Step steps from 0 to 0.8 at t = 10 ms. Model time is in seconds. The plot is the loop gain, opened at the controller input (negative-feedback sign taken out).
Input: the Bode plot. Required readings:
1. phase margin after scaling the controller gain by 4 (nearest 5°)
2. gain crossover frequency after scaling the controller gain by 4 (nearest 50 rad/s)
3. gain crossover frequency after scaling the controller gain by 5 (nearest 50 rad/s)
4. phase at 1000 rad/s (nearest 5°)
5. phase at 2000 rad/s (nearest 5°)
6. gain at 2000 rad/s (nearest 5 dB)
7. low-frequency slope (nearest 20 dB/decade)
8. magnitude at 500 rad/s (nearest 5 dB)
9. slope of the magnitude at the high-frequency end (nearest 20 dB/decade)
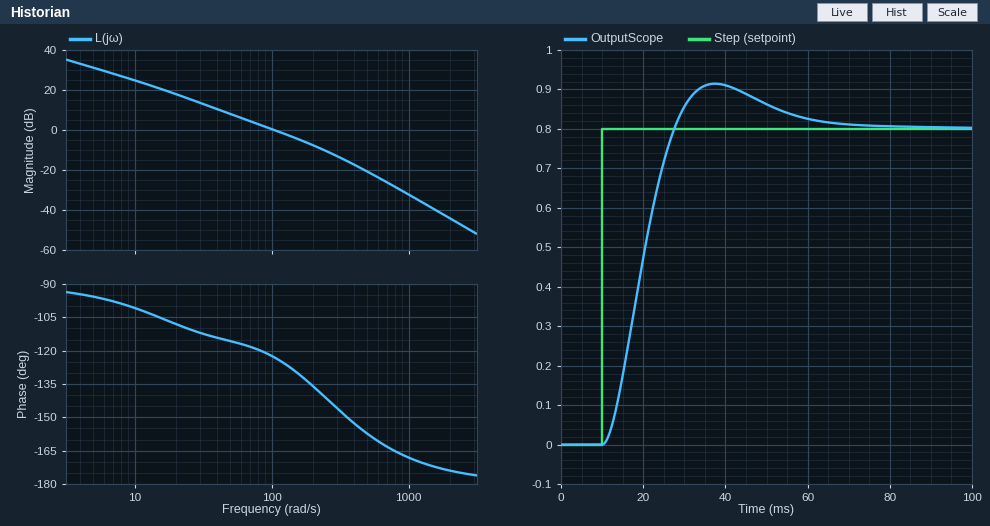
35°
300 rad/s
300 rad/s
-170°
-175°
-45 dB
-20 dB/decade
-20 dB
-40 dB/decade
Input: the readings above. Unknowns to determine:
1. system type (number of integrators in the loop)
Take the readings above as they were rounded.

1
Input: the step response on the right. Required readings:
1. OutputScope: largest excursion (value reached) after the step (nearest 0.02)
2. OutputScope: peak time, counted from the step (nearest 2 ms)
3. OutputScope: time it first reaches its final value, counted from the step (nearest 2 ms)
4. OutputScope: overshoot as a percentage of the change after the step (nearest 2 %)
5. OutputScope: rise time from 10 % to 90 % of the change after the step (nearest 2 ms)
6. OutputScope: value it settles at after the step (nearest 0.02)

0.92
28 ms
18 ms
14 %
12 ms
0.80
